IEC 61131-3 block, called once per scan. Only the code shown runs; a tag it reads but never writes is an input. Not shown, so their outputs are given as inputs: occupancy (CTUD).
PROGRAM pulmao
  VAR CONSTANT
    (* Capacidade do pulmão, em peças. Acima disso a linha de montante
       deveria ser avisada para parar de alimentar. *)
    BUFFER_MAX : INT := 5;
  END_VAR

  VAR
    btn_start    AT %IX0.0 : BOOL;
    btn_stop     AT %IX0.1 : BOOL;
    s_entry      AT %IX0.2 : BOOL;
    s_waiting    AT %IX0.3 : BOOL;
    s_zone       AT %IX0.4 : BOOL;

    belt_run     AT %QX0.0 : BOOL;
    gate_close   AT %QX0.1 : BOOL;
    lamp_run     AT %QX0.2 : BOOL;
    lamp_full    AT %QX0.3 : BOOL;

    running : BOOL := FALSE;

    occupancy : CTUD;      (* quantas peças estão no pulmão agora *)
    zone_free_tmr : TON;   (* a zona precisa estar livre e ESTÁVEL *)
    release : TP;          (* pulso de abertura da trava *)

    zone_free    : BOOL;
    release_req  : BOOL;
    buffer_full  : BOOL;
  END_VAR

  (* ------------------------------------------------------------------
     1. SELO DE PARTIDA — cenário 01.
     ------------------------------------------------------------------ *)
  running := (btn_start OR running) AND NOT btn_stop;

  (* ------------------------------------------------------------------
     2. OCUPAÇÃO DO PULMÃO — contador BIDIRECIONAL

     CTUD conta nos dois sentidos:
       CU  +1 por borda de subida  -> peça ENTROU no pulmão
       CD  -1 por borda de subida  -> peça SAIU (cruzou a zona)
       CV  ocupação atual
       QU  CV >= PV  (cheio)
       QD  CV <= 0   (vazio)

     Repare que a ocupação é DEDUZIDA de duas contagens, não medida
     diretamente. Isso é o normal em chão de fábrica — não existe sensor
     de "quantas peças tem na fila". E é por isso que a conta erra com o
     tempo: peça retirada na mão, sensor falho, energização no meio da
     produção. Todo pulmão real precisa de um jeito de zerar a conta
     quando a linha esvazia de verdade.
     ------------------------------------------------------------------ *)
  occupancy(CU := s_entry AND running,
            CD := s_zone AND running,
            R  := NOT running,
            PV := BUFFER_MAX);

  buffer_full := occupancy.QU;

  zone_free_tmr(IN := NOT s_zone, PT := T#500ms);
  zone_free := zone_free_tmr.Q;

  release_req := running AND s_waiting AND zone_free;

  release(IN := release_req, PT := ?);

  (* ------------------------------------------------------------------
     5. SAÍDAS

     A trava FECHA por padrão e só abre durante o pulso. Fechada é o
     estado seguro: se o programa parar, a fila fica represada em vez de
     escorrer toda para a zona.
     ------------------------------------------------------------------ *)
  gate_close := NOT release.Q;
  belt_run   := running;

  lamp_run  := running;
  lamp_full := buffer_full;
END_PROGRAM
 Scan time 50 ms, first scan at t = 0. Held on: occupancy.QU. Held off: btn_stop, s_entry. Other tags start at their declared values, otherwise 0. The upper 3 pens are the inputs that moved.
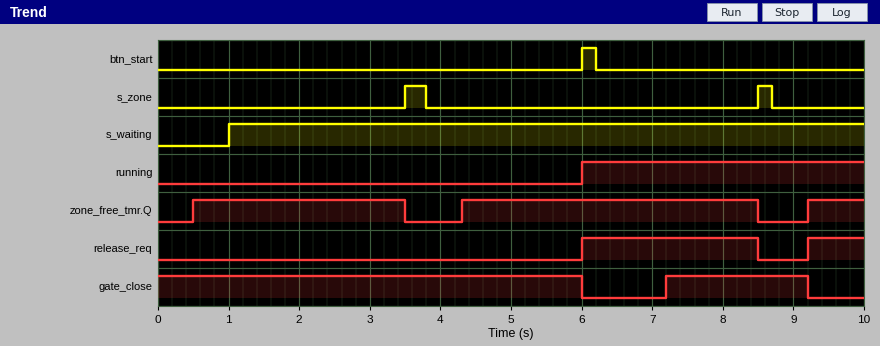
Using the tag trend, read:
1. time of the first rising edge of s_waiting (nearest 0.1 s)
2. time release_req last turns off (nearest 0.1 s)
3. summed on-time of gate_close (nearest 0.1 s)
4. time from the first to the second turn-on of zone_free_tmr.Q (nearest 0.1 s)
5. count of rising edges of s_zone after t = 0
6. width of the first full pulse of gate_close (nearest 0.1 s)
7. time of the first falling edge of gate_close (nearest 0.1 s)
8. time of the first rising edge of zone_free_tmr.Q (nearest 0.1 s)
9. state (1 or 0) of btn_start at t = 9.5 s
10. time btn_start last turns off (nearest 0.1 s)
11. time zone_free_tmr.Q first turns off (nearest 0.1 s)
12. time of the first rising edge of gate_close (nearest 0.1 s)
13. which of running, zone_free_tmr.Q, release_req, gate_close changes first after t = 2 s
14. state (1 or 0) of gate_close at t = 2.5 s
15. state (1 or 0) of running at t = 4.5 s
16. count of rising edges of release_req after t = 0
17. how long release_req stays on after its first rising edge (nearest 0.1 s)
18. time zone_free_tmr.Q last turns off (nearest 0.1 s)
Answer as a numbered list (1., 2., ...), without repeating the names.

1. 1.0 s
2. 8.5 s
3. 8.0 s
4. 3.8 s
5. 2
6. 2.0 s
7. 6.0 s
8. 0.5 s
9. 0
10. 6.2 s
11. 3.5 s
12. 7.2 s
13. zone_free_tmr.Q
14. 1
15. 0
16. 2
17. 2.5 s
18. 8.5 s
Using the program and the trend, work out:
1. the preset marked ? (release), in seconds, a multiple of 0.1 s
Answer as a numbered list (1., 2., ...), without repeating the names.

1. 1.2 s
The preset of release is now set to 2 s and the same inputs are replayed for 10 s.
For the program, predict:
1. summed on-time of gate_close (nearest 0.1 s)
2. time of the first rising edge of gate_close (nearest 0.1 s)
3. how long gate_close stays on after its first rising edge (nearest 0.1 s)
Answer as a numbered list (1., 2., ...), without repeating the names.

1. 7.2 s
2. 8.0 s
3. 1.2 s
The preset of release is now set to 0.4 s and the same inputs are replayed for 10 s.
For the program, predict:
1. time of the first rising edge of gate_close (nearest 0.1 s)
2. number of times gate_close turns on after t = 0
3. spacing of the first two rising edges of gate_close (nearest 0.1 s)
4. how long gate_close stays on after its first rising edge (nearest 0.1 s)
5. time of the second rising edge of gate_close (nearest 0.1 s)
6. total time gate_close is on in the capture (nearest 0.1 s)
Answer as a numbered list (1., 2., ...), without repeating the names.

1. 6.4 s
2. 2
3. 3.2 s
4. 2.8 s
5. 9.6 s
6. 9.2 s
